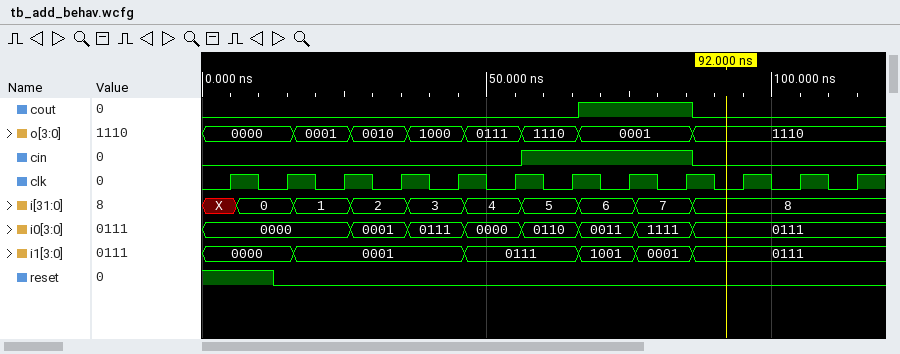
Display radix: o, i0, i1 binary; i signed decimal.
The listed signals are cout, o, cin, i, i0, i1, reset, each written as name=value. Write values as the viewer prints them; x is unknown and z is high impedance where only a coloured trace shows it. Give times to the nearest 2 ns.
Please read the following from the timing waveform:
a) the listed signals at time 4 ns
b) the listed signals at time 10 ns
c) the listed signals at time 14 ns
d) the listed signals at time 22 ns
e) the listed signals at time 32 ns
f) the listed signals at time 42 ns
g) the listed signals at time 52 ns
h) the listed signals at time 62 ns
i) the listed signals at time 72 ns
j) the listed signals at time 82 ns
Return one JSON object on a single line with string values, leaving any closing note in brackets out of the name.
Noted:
{"the listed signals at time 4 ns": "cout=0, o=0000, cin=0, i=X, i0=0000, i1=0000, reset=1", "the listed signals at time 10 ns": "cout=0, o=0000, cin=0, i=0, i0=0000, i1=0000, reset=1", "the listed signals at time 14 ns": "cout=0, o=0000, cin=0, i=0, i0=0000, i1=0000, reset=0", "the listed signals at time 22 ns": "cout=0, o=0001, cin=0, i=1, i0=0000, i1=0001, reset=0", "the listed signals at time 32 ns": "cout=0, o=0010, cin=0, i=2, i0=0001, i1=0001, reset=0", "the listed signals at time 42 ns": "cout=0, o=1000, cin=0, i=3, i0=0111, i1=0001, reset=0", "the listed signals at time 52 ns": "cout=0, o=0111, cin=0, i=4, i0=0000, i1=0111, reset=0", "the listed signals at time 62 ns": "cout=0, o=1110, cin=1, i=5, i0=0110, i1=0111, reset=0", "the listed signals at time 72 ns": "cout=1, o=0001, cin=1, i=6, i0=0011, i1=1001, reset=0", "the listed signals at time 82 ns": "cout=1, o=0001, cin=1, i=7, i0=1111, i1=0001, reset=0"}
